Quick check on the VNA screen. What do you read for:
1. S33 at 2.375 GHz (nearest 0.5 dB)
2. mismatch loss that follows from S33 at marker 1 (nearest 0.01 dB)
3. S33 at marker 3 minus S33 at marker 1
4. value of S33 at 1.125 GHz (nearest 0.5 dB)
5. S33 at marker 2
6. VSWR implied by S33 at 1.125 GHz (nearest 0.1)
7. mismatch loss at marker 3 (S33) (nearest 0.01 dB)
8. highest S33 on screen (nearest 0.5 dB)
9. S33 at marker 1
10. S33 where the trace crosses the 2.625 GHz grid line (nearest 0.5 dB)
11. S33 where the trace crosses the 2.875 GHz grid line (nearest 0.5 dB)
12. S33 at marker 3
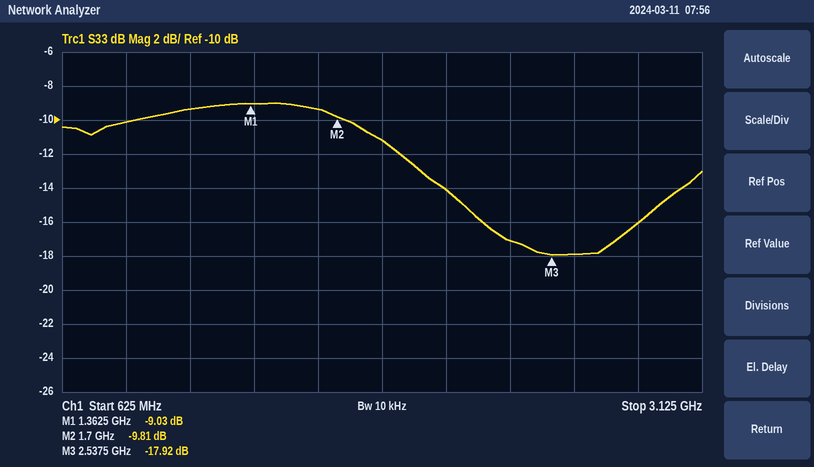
-17.0 dB
0.58 dB
-8.89 dB
-9.5 dB
-9.81 dB
2.0
0.07 dB
-9.0 dB
-9.03 dB
-18.0 dB
-16.0 dB
-17.92 dB
